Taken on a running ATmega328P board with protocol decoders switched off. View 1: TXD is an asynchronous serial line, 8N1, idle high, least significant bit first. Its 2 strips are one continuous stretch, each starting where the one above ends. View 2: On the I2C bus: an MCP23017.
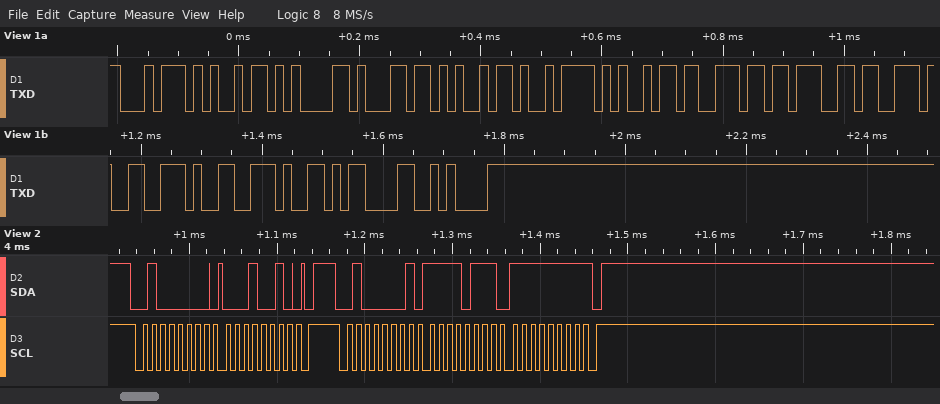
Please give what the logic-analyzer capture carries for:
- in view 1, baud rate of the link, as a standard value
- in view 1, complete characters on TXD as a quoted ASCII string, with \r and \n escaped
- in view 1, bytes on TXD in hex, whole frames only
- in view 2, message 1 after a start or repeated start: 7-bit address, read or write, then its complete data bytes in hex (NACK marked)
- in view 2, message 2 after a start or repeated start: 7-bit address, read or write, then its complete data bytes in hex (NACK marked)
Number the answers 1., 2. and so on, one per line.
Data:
1. 74880 baud
2. "tializing...\r\n"
3. 74 69 61 6C 69 7A 69 6E 67 2E 2E 2E 0D 0A
4. 0x20 write: 12
5. 0x20 read: F7 FF NACK
